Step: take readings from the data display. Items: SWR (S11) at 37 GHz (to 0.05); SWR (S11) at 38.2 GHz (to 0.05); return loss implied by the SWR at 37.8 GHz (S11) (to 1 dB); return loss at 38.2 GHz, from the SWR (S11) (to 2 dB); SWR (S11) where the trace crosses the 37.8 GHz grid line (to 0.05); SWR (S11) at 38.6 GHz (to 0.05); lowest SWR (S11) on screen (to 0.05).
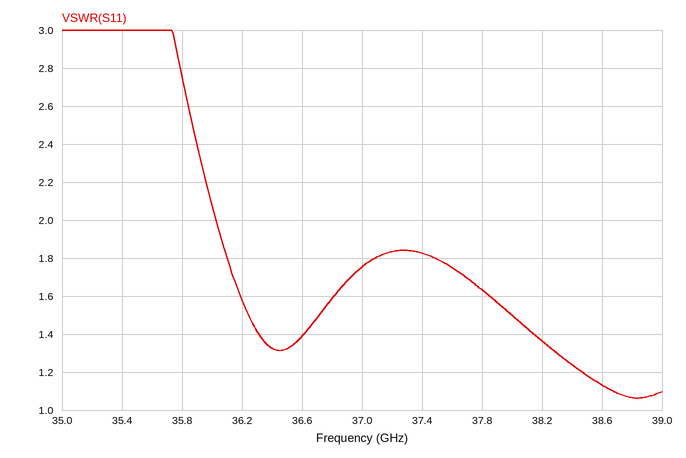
1.75
1.35
12 dB
16 dB
1.65
1.15
1.05
